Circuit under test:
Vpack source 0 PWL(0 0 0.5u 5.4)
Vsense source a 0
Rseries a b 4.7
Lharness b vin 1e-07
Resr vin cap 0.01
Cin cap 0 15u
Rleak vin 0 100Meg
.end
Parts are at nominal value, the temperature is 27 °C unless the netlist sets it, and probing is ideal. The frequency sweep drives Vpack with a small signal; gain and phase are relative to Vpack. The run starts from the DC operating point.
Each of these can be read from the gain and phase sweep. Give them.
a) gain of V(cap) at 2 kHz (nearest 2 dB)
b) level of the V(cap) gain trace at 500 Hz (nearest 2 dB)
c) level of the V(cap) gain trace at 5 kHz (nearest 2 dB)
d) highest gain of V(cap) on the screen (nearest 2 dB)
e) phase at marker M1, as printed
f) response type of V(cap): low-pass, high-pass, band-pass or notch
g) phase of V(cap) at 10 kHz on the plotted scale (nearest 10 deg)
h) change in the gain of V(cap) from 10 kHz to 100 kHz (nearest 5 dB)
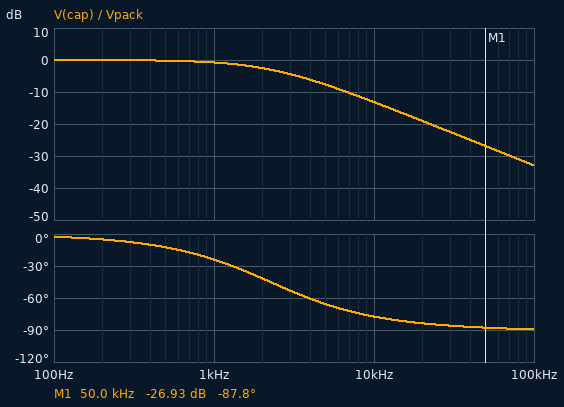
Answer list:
-2 dB
0 dB
-8 dB
0 dB
-87.8 deg
low-pass
-80 deg
-20 dB
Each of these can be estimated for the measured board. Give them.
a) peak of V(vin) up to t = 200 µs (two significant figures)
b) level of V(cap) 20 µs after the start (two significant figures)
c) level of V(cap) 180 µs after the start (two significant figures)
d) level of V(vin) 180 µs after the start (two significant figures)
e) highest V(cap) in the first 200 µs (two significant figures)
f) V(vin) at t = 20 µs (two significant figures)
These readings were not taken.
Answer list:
5.1 V
1.3 V
5.0 V
5.0 V
5.1 V
1.3 V
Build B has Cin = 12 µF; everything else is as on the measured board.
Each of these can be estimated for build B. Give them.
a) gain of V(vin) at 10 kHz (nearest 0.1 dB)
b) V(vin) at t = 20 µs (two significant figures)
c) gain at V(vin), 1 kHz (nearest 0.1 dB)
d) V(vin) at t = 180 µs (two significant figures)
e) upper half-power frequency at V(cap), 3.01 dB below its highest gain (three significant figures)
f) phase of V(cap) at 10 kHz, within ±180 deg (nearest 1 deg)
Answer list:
-11.3 dB
1.6 V
-0.5 dB
5.2 V
2.82 kHz
-74 deg
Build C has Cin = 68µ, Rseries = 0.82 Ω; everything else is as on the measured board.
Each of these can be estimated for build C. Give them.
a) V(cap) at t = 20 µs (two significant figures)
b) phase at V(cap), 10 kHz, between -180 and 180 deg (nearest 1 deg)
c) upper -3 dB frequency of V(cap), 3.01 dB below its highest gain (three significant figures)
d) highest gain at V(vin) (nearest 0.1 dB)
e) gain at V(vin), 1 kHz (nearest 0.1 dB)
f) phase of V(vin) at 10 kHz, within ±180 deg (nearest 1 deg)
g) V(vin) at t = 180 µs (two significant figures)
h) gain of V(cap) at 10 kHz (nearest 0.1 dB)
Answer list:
1.6 V
-75 deg
2.83 kHz
0 dB
-0.5 dB
-72 deg
5.2 V
-11.3 dB
